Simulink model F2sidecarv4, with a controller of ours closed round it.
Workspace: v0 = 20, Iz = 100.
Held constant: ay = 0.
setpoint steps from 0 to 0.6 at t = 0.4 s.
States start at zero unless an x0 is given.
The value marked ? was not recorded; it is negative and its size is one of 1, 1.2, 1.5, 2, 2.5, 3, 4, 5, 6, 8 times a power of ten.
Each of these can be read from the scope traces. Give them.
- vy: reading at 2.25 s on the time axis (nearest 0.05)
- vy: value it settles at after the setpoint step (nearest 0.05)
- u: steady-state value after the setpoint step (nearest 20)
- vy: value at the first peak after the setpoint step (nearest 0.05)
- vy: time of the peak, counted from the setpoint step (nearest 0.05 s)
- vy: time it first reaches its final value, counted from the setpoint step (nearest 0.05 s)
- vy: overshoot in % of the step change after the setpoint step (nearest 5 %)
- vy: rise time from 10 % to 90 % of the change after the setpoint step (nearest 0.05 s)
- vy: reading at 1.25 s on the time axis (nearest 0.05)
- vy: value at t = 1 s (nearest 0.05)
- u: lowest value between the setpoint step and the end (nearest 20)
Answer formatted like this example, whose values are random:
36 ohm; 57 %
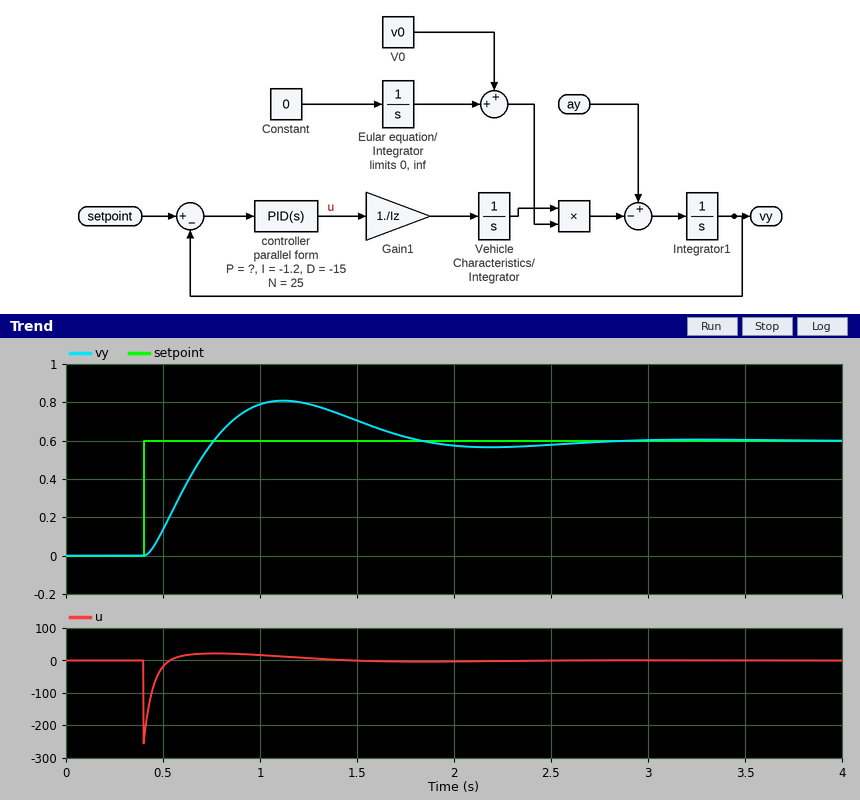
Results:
0.55; 0.60; 0; 0.80; 0.70 s; 0.35 s; 35 %; 0.25 s; 0.80; 0.80; -260
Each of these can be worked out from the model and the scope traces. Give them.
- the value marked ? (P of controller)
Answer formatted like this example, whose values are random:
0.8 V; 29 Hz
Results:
-50
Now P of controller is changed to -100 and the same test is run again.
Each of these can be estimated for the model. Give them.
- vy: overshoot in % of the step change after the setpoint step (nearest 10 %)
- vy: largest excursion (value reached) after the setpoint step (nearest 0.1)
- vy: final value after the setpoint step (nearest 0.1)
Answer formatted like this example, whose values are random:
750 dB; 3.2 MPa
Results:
50 %; 0.9; 0.6
